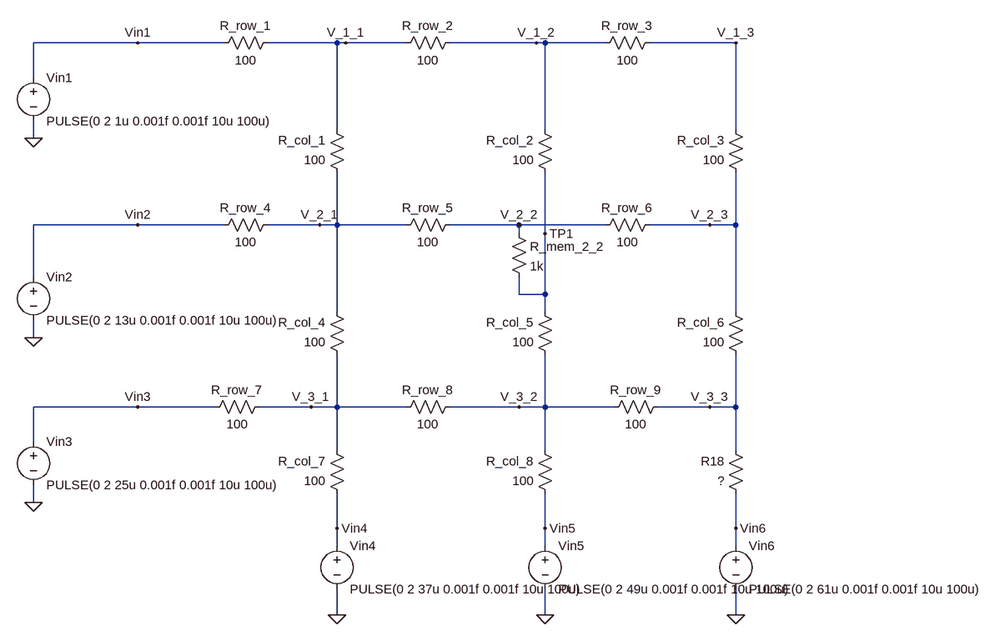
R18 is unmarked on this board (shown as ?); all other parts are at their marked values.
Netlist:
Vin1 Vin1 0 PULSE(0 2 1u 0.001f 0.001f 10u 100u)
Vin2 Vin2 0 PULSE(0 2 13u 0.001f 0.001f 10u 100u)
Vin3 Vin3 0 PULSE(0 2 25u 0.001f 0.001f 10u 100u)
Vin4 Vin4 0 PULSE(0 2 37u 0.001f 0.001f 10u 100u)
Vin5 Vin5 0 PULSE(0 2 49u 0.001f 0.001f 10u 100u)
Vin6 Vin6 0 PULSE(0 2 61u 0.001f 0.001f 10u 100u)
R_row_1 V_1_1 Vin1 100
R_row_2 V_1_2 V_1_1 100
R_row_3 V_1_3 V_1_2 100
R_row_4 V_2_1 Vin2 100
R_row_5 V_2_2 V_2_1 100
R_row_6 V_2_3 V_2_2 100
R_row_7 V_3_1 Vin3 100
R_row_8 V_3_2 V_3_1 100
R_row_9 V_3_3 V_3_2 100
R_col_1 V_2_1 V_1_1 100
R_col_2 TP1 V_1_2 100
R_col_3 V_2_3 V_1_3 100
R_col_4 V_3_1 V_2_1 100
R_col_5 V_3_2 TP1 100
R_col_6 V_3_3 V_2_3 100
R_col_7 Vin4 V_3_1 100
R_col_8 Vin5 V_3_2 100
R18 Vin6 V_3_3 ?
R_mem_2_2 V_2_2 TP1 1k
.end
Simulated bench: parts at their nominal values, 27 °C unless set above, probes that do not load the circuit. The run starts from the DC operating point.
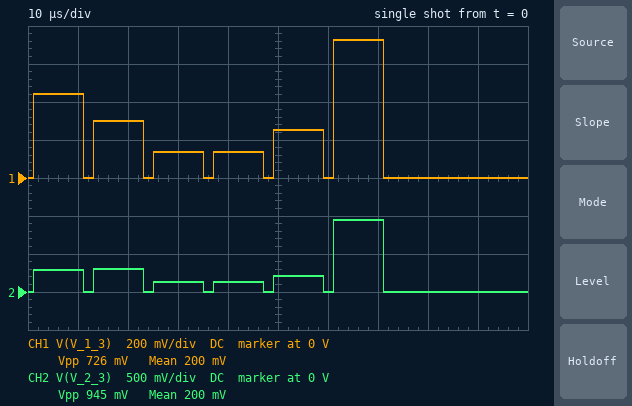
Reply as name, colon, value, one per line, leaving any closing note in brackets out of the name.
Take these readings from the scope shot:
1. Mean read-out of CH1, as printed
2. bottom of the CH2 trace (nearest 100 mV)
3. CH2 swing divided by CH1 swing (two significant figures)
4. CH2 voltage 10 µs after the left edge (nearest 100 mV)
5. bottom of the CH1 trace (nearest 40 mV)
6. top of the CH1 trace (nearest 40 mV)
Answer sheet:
Mean read-out of CH1, as printed: 200 mV
bottom of the CH2 trace: 0 V
CH2 swing divided by CH1 swing: 1.3
CH2 voltage 10 µs after the left edge: 300 mV
bottom of the CH1 trace: 0 V
top of the CH1 trace: 720 mV
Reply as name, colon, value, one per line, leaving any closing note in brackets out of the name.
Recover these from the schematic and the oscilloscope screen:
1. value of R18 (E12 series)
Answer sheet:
value of R18: 33 Ω
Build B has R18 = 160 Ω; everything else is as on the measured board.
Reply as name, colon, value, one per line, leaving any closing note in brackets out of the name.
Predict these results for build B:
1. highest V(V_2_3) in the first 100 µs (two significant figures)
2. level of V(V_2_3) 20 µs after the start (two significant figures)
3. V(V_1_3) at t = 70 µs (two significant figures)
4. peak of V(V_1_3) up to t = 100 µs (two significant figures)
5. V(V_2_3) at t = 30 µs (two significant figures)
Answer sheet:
highest V(V_2_3) in the first 100 µs: 480 mV
level of V(V_2_3) 20 µs after the start: 390 mV
V(V_1_3) at t = 70 µs: 370 mV
peak of V(V_1_3) up to t = 100 µs: 500 mV
V(V_2_3) at t = 30 µs: 190 mV
